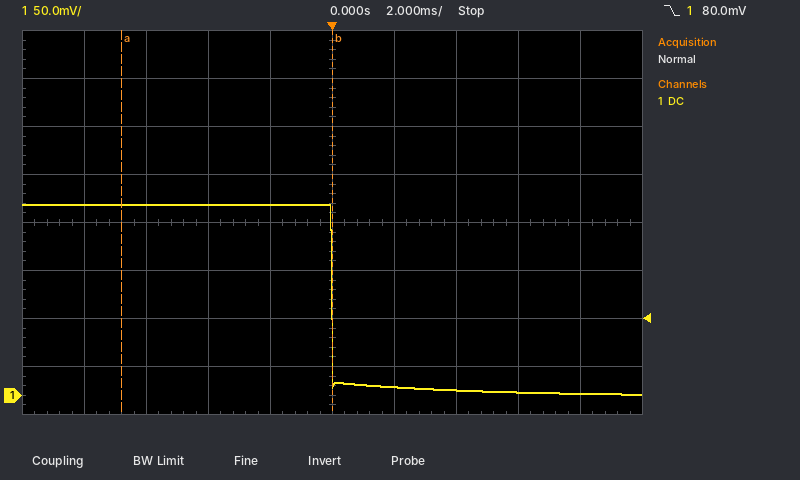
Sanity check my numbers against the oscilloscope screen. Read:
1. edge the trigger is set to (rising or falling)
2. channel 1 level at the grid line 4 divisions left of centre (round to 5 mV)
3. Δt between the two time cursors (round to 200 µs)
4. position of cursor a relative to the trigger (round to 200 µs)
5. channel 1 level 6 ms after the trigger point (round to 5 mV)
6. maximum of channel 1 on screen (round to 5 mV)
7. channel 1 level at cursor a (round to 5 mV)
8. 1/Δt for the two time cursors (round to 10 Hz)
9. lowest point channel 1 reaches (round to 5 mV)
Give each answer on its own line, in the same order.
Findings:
falling
200 mV
6.8 ms
-6.8 ms
5 mV
200 mV
200 mV
150 Hz
0 mV
